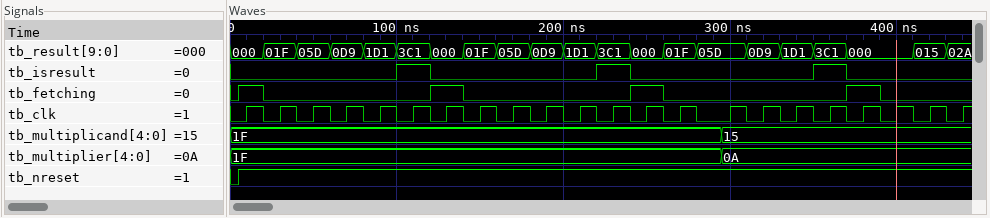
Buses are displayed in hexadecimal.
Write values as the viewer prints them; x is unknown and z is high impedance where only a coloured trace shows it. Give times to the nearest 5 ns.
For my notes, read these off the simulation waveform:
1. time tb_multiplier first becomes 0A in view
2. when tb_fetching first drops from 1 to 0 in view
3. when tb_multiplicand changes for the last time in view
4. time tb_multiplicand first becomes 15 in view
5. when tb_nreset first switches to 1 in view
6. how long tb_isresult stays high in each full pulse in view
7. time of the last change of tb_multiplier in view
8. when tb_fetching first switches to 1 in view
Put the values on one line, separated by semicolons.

295 ns; 20 ns; 295 ns; 295 ns; 5 ns; 20 ns, 20 ns, 20 ns; 295 ns; 5 ns
